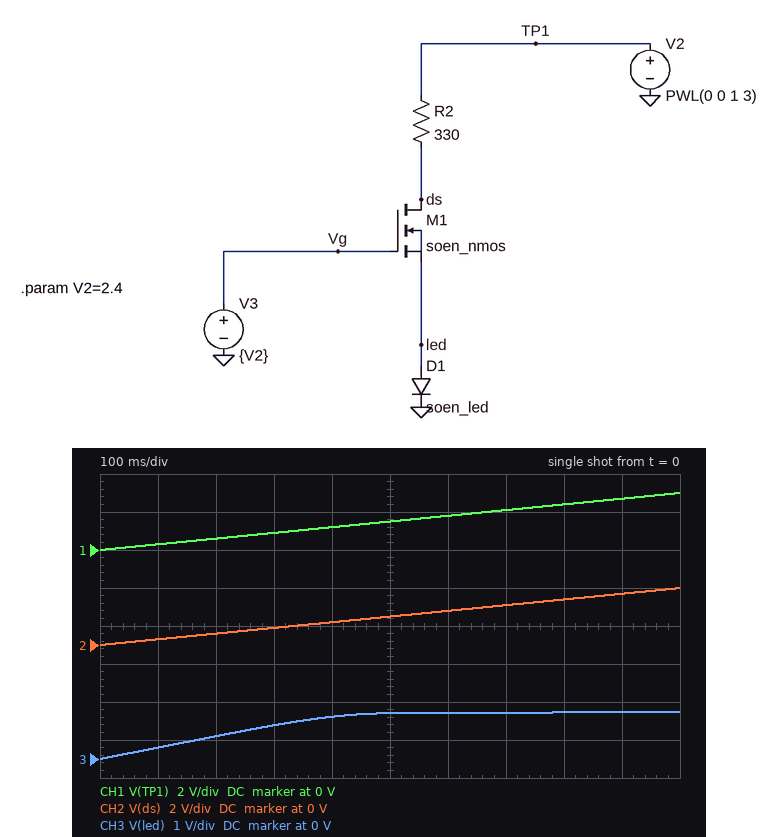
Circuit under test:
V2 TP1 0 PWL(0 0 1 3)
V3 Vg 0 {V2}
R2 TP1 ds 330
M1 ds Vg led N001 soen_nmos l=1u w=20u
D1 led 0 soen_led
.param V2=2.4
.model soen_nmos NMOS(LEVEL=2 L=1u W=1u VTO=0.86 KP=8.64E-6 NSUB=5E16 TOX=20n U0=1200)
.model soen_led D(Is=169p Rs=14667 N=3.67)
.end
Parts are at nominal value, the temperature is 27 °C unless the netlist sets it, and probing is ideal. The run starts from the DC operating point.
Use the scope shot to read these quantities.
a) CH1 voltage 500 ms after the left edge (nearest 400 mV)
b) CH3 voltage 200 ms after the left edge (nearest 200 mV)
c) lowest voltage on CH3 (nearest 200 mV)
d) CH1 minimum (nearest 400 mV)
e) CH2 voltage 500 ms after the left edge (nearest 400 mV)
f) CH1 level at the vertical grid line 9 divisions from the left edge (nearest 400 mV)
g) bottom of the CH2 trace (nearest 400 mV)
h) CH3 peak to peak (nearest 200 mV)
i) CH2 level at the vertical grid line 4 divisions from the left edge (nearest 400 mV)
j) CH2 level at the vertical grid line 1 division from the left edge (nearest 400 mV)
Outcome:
1.6 V
600 mV
0 V
0 V
1.6 V
2.8 V
0 V
1.2 V
1.2 V
400 mV
